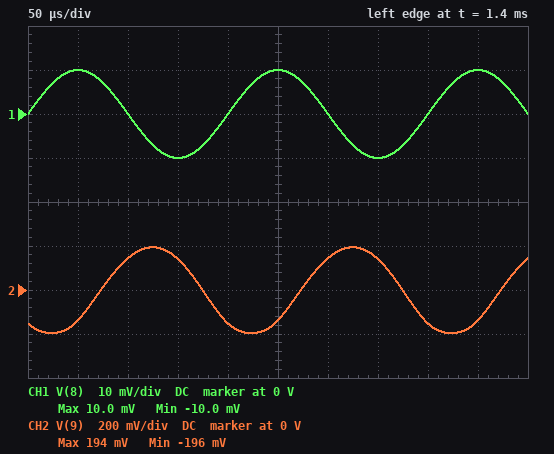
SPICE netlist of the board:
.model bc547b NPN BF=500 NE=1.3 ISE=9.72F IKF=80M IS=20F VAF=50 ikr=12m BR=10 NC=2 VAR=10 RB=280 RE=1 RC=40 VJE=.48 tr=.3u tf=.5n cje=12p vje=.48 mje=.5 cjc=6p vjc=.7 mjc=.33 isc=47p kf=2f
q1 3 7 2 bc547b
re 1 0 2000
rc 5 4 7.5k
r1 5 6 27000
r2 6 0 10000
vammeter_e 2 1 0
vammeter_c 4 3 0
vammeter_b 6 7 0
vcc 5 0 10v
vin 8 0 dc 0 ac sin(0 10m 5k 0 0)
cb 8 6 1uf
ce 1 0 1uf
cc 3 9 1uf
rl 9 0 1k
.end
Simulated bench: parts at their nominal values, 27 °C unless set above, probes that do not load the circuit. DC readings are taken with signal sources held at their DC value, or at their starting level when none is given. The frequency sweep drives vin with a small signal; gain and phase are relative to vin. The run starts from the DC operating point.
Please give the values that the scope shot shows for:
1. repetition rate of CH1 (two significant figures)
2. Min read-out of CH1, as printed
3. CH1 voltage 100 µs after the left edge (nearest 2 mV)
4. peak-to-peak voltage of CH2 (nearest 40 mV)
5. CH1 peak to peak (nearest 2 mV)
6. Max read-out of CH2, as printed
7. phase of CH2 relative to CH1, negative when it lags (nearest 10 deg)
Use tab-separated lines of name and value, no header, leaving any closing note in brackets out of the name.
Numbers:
repetition rate of CH1	5.0 kHz
Min read-out of CH1, as printed	-10.0 mV
CH1 voltage 100 µs after the left edge	0 V
peak-to-peak voltage of CH2	400 mV
CH1 peak to peak	20 mV
Max read-out of CH2, as printed	194 mV
phase of CH2 relative to CH1, negative when it lags	-130 deg
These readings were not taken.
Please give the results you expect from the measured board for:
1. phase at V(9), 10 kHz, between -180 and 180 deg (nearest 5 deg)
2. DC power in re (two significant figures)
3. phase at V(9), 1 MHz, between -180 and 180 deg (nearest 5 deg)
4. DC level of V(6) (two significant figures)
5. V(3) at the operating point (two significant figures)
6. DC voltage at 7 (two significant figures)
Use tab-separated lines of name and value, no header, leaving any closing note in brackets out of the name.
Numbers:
phase at V(9), 10 kHz, between -180 and 180 deg	-150 deg
DC power in re	2.1 mW
phase at V(9), 1 MHz, between -180 and 180 deg	150 deg
DC level of V(6)	2.7 V
V(3) at the operating point	2.4 V
DC voltage at 7	2.7 V
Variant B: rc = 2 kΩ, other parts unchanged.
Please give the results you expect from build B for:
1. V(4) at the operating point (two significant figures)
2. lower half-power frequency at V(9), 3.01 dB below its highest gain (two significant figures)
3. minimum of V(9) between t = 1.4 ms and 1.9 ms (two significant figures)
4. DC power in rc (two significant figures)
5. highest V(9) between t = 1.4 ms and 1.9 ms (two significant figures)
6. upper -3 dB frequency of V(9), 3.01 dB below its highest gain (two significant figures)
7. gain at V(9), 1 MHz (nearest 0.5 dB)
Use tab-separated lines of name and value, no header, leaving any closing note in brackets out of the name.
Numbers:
V(4) at the operating point	8.0 V
lower half-power frequency at V(9), 3.01 dB below its highest gain	5.8 kHz
minimum of V(9) between t = 1.4 ms and 1.9 ms	-160 mV
DC power in rc	2.1 mW
highest V(9) between t = 1.4 ms and 1.9 ms	150 mV
upper -3 dB frequency of V(9), 3.01 dB below its highest gain	4.4 MHz
gain at V(9), 1 MHz	27.5 dB
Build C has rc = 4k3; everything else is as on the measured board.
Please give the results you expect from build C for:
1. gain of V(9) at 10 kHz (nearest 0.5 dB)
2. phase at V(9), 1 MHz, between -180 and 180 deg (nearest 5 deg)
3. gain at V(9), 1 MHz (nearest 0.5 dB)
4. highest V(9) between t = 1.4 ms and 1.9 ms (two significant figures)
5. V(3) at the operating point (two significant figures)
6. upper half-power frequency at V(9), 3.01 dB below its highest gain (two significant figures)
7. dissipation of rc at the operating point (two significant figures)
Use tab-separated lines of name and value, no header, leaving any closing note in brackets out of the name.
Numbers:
gain of V(9) at 10 kHz	28.0 dB
phase at V(9), 1 MHz, between -180 and 180 deg	165 deg
gain at V(9), 1 MHz	29.0 dB
highest V(9) between t = 1.4 ms and 1.9 ms	180 mV
V(3) at the operating point	5.6 V
upper half-power frequency at V(9), 3.01 dB below its highest gain	3.5 MHz
dissipation of rc at the operating point	4.4 mW
